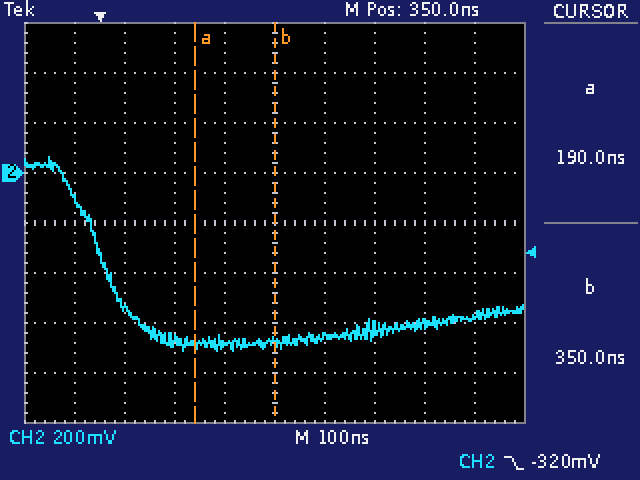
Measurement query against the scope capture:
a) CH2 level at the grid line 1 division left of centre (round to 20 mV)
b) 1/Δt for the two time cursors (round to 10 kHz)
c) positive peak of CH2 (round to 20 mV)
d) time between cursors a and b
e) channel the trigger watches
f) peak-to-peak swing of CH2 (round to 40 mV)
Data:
-680 mV
6.25 MHz
60 mV
160 ns
CH2
760 mV
